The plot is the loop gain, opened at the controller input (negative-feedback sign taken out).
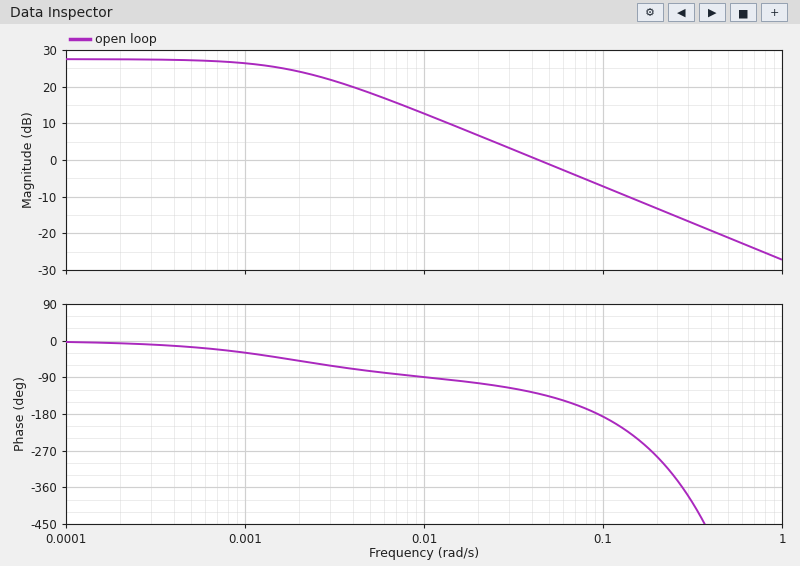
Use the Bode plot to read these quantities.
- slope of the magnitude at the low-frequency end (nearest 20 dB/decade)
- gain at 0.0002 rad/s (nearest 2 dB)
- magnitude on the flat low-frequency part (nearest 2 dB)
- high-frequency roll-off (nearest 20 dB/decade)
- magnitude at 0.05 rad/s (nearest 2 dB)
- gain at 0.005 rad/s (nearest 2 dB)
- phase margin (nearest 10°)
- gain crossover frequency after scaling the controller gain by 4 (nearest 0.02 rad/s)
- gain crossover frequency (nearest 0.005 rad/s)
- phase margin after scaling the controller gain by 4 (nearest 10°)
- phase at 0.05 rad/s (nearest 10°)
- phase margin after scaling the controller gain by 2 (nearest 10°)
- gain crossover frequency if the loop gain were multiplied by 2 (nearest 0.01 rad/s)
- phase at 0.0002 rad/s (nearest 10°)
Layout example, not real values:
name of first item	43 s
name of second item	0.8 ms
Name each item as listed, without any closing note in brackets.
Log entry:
slope of the magnitude at the low-frequency end	0 dB/decade
gain at 0.0002 rad/s	28 dB
magnitude on the flat low-frequency part	28 dB
high-frequency roll-off	-20 dB/decade
magnitude at 0.05 rad/s	-2 dB
gain at 0.005 rad/s	18 dB
phase margin	50°
gain crossover frequency after scaling the controller gain by 4	0.18 rad/s
gain crossover frequency	0.045 rad/s
phase margin after scaling the controller gain by 4	-80°
phase at 0.05 rad/s	-140°
phase margin after scaling the controller gain by 2	10°
gain crossover frequency if the loop gain were multiplied by 2	0.09 rad/s
phase at 0.0002 rad/s	-10°
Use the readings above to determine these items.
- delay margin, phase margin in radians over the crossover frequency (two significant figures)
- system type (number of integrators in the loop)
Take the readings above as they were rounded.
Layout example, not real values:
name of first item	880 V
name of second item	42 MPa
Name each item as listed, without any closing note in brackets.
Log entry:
delay margin, phase margin in radians over the crossover frequency	19 s
system type	0
